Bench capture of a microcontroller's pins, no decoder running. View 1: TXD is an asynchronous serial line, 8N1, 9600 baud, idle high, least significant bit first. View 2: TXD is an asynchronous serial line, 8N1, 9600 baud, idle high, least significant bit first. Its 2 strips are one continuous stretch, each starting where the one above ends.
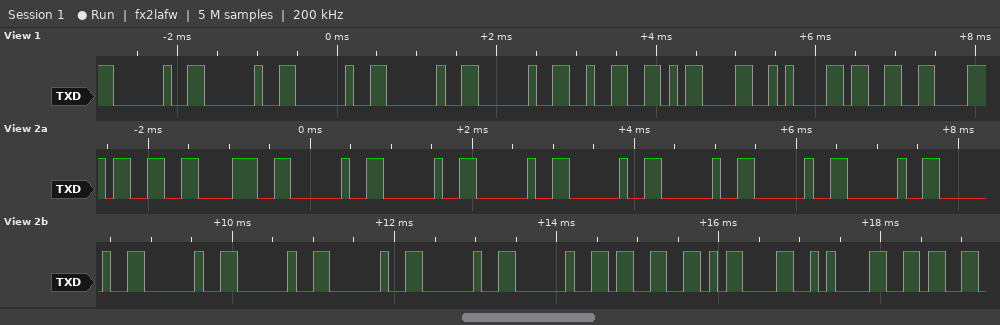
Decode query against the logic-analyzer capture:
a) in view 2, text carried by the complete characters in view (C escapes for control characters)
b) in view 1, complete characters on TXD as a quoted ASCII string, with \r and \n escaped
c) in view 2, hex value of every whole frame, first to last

"38             3\r\n6"
"     2\r\n3"
33 38 20 20 20 20 20 20 20 20 20 20 20 20 20 33 0D 0A 36
